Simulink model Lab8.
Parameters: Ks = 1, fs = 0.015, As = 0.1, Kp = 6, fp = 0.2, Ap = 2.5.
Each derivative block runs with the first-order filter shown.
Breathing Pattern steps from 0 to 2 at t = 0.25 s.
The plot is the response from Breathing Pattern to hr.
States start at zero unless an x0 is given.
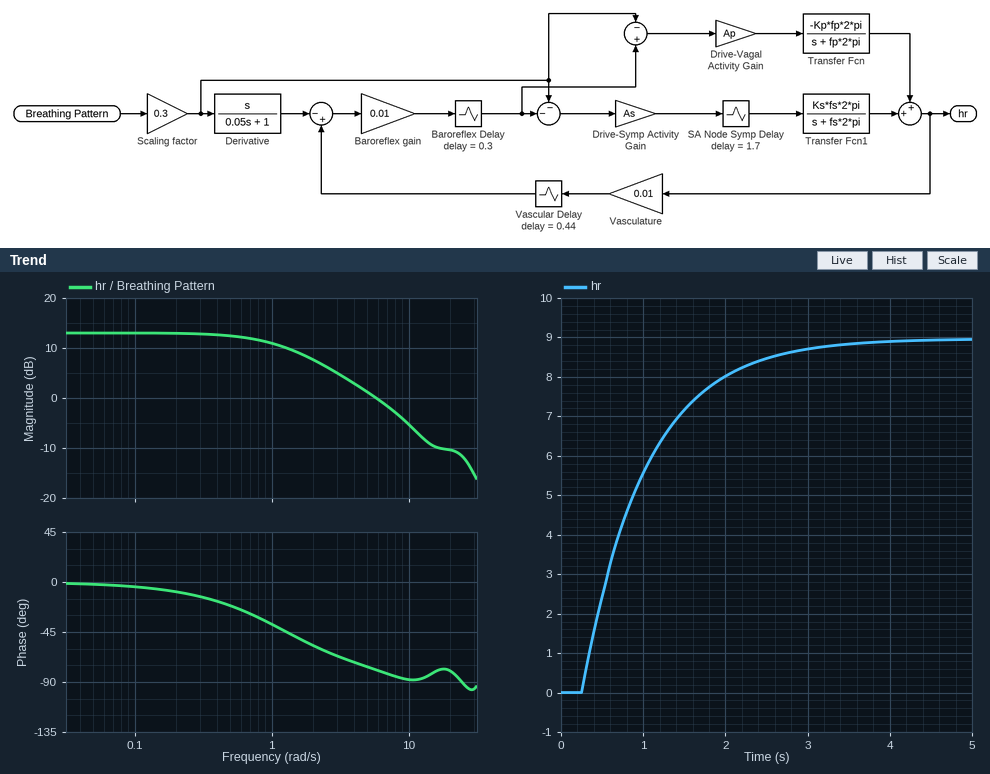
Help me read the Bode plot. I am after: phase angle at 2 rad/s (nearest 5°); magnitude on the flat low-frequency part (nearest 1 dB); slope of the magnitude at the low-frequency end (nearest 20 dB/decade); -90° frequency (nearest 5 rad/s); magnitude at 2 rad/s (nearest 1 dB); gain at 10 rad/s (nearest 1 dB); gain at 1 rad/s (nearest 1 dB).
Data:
-55°
13 dB
0 dB/decade
25 rad/s
8 dB
-5 dB
11 dB
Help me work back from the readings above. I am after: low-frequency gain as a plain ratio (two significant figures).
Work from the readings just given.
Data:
4.5
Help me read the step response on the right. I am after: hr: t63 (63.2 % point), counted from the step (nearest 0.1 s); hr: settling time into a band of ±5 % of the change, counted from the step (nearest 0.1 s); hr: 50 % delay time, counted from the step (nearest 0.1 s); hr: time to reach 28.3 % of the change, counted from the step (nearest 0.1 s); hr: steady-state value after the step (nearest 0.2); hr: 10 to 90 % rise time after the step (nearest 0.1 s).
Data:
0.8 s
2.3 s
0.5 s
0.3 s
9.0
1.7 s
